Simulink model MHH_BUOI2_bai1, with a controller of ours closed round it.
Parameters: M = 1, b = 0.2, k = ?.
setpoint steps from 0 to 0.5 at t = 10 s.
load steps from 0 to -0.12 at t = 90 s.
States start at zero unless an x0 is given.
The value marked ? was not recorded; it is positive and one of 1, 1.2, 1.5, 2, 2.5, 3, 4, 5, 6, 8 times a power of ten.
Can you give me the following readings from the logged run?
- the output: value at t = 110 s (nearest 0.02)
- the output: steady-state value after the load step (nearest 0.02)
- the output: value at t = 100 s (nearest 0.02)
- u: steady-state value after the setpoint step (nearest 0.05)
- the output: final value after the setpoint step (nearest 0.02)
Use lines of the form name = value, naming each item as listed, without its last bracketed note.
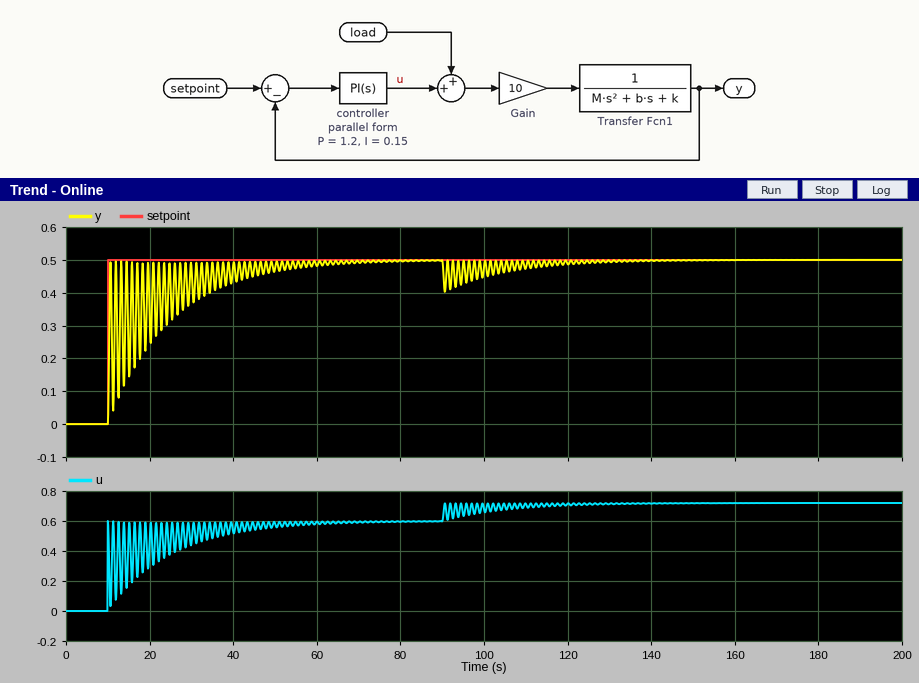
the output: value at t = 110 s = 0.48
the output: steady-state value after the load step = 0.50
the output: value at t = 100 s = 0.48
u: steady-state value after the setpoint step = 0.60
the output: final value after the setpoint step = 0.50
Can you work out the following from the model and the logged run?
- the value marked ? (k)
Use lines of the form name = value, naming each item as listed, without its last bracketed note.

the value marked ? = 12
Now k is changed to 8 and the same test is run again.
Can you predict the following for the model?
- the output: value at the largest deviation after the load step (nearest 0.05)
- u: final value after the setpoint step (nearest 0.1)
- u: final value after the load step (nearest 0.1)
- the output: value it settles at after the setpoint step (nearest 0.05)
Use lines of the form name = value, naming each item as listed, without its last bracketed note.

the output: value at the largest deviation after the load step = 0.40
u: final value after the setpoint step = 0.4
u: final value after the load step = 0.5
the output: value it settles at after the setpoint step = 0.50
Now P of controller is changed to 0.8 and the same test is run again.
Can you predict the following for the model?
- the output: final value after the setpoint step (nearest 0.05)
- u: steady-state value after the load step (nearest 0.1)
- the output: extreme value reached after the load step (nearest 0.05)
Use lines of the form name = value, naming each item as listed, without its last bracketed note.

the output: final value after the setpoint step = 0.50
u: steady-state value after the load step = 0.7
the output: extreme value reached after the load step = 0.40
